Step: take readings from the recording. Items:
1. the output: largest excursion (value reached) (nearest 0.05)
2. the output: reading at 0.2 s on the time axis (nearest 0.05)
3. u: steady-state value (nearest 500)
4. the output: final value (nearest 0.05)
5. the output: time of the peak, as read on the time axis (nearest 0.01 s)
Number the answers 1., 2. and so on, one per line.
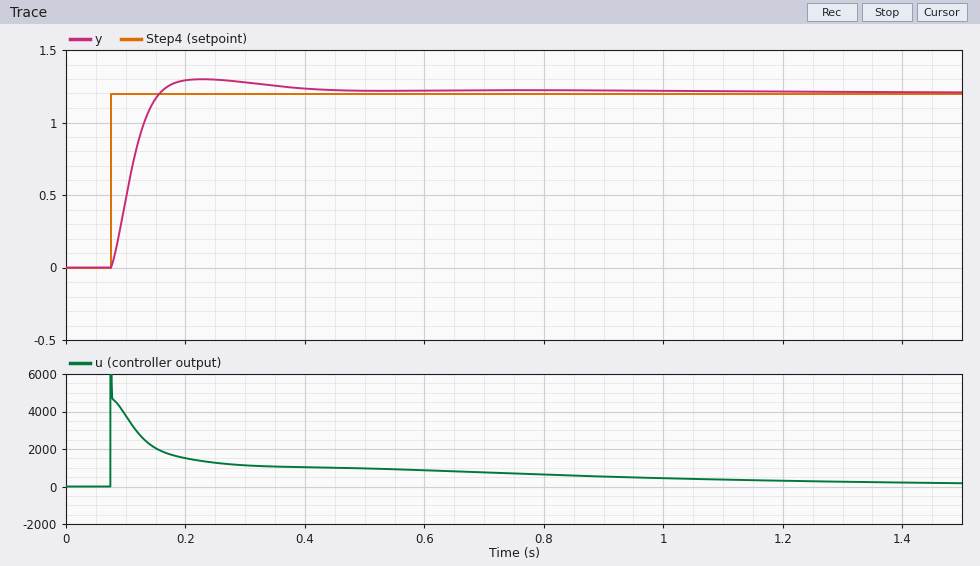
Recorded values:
1. 1.30
2. 1.30
3. 0
4. 1.20
5. 0.23 s
